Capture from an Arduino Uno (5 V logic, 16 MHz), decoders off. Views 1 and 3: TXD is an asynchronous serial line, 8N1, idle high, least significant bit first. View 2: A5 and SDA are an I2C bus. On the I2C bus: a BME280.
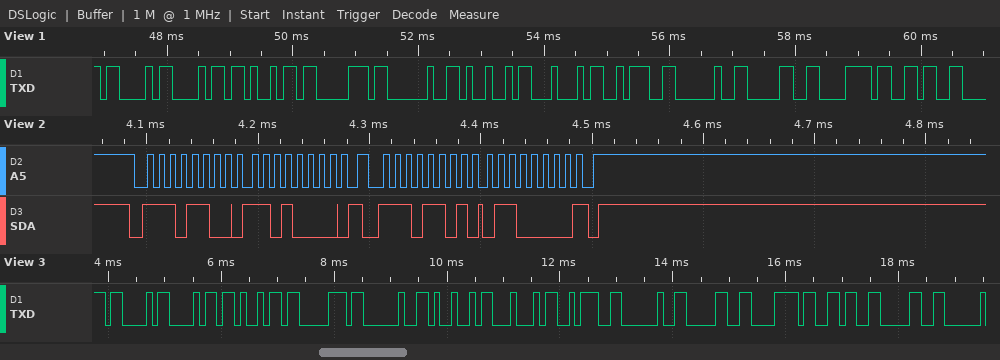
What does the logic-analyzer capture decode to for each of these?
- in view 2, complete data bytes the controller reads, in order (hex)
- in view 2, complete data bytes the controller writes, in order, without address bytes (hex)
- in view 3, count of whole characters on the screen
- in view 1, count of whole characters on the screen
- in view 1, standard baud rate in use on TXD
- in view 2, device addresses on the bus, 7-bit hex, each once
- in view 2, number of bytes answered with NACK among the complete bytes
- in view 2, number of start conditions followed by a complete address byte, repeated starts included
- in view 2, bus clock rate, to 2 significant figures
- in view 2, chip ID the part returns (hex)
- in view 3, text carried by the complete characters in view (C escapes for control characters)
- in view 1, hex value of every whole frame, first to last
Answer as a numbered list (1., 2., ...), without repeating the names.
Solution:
1. 60
2. D0
3. 13
4. 12
5. 9600 baud
6. 0x76
7. 1
8. 2
9. 100 kHz
10. 0x60
11. "Chip ID: 0x60"
12. 43 68 69 70 20 49 44 3A 20 30 78 36
